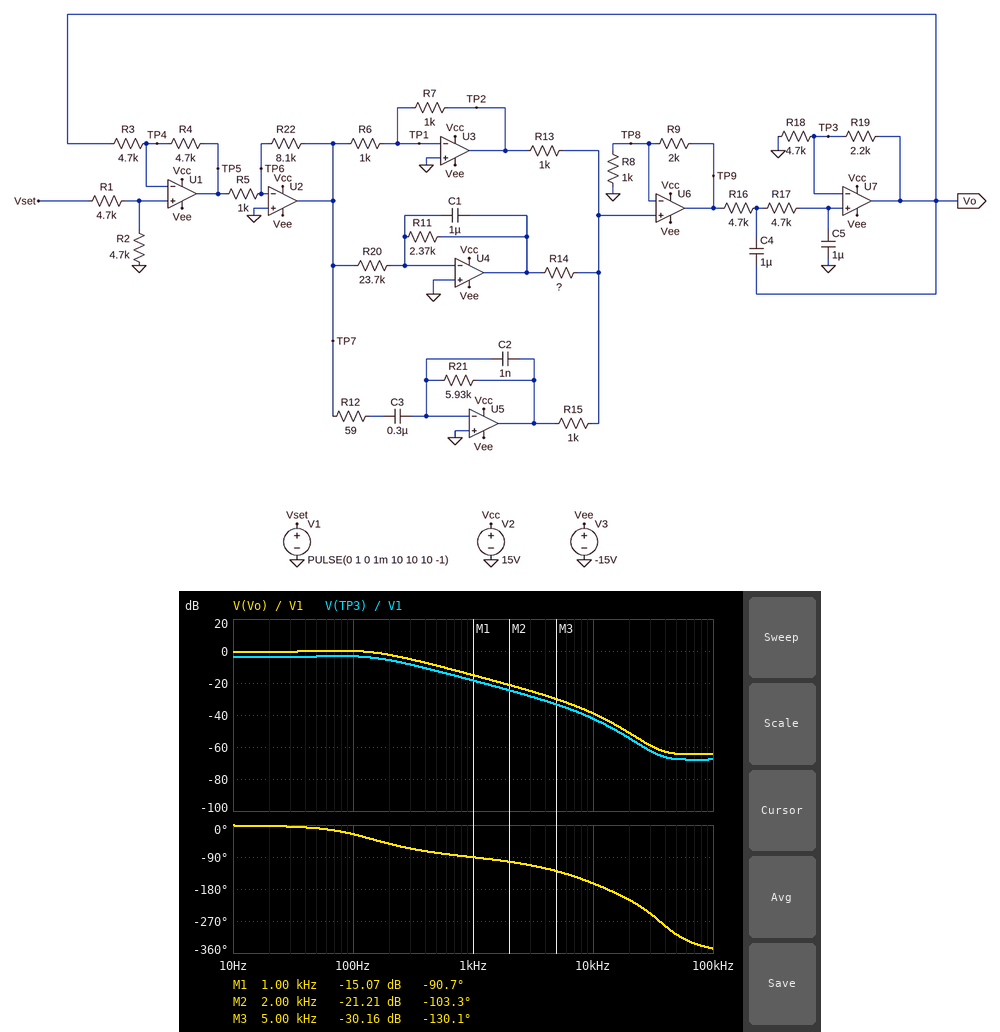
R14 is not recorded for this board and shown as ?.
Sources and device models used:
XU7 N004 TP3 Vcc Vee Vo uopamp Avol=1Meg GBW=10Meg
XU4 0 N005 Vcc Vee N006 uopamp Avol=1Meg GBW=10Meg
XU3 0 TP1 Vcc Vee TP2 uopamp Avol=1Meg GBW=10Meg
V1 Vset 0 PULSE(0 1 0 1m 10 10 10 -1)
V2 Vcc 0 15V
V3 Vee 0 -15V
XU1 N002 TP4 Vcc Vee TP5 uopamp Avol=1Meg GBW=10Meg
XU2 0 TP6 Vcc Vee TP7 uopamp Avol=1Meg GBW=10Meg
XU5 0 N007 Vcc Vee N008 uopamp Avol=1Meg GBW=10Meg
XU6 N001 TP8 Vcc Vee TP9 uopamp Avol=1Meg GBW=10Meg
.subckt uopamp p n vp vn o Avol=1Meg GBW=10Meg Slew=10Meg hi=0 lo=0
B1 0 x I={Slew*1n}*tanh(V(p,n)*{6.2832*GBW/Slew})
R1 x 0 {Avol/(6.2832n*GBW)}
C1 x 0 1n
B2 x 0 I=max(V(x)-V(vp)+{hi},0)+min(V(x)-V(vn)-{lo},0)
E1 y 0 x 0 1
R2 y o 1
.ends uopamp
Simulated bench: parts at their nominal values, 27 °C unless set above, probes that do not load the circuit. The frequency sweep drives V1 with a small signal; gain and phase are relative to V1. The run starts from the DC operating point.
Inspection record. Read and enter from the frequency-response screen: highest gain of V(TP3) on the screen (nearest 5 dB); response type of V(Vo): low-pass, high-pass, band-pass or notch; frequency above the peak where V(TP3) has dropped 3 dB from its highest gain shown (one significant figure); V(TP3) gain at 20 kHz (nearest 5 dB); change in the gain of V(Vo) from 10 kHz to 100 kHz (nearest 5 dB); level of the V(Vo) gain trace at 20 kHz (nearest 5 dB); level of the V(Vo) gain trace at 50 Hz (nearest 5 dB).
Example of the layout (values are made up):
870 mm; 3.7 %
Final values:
-5 dB; low-pass; 200 Hz; -55 dB; -25 dB; -50 dB; 0 dB
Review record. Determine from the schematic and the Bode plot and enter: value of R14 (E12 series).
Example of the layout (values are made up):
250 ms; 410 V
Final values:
1.5 kΩ
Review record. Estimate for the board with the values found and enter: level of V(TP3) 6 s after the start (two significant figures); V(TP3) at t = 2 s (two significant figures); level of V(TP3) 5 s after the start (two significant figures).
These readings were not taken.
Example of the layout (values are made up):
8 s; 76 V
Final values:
640 mV; 640 mV; 640 mV
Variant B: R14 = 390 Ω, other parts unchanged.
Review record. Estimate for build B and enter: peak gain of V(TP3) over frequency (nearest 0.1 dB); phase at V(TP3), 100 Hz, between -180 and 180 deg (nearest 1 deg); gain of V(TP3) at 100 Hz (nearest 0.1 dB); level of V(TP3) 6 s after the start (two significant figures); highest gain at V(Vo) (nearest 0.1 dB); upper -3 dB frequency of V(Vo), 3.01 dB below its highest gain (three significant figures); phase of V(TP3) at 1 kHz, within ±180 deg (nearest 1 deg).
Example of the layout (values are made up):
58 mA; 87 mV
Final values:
-3.1 dB; -44 deg; -3.9 dB; 620 mV; 0.2 dB; 142 Hz; -95 deg
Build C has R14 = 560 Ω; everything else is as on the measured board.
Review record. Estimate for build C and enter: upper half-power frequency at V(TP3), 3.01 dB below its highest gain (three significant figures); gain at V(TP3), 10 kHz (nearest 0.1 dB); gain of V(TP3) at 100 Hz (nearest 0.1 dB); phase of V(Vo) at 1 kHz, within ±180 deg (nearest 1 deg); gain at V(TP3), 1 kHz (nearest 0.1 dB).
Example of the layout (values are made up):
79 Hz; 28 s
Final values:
164 Hz; -45.4 dB; -3.6 dB; -94 deg; -21.5 dB
